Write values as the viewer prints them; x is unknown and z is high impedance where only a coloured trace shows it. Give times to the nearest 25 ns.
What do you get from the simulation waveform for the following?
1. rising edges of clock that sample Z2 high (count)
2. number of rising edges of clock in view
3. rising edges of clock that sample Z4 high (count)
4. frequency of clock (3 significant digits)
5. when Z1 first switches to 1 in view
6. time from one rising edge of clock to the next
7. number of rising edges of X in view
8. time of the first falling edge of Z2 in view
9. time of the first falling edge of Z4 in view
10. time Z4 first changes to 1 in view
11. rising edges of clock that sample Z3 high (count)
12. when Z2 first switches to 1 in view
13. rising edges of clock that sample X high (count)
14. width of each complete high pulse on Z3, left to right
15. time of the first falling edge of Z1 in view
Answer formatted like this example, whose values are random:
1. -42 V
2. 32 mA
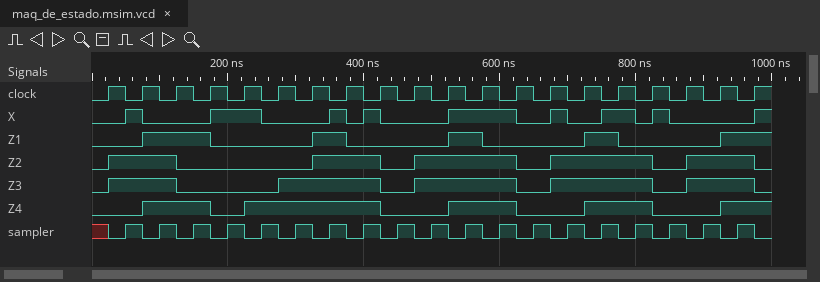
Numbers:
1. 12
2. 20
3. 11
4. 20.0 MHz
5. 75 ns
6. 50 ns
7. 9
8. 125 ns
9. 175 ns
10. 75 ns
11. 13
12. 25 ns
13. 7
14. 100 ns, 150 ns, 150 ns, 150 ns, 100 ns
15. 175 ns
